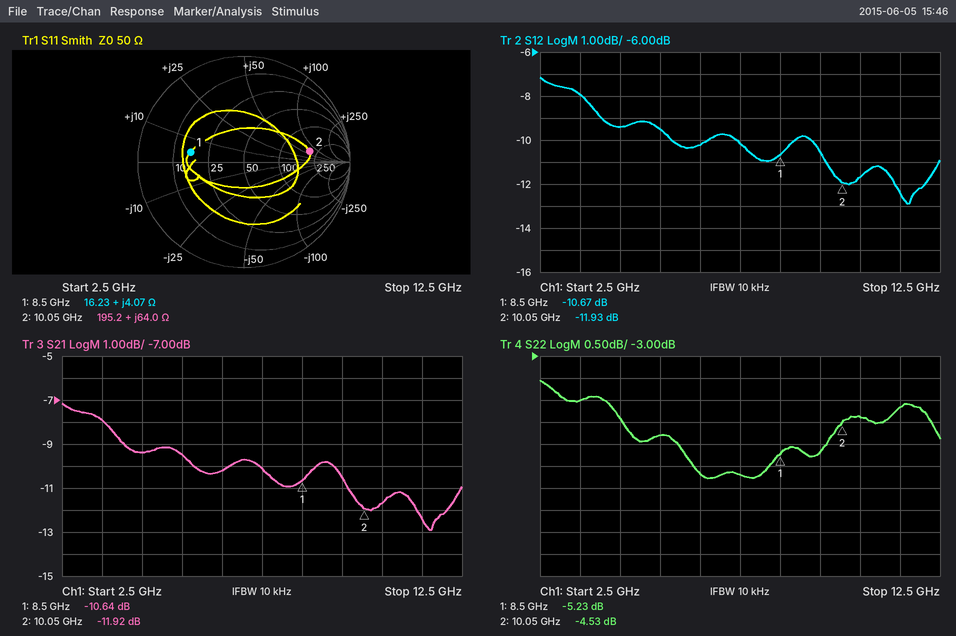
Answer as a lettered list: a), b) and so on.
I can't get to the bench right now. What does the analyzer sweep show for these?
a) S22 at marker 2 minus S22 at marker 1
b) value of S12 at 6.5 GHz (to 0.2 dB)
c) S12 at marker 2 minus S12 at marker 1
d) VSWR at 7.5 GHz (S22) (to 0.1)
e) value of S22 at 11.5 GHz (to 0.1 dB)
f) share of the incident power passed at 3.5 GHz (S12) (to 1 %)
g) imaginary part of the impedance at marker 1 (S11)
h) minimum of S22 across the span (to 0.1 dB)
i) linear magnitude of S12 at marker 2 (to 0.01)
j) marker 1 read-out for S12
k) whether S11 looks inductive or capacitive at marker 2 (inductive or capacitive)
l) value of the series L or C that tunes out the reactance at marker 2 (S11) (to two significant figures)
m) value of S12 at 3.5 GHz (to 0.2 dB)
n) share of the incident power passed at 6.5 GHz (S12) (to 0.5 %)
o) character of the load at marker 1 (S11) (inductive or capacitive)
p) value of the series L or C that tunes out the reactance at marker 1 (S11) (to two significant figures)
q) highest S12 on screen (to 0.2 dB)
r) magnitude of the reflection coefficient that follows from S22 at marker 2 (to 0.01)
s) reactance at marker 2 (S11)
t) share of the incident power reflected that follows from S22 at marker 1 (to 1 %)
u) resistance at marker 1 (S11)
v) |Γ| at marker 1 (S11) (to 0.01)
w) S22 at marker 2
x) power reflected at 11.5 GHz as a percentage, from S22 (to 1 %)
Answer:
a) 0.70 dB
b) -10.2 dB
c) -1.26 dB
d) 3.2
e) -4.2 dB
f) 16 %
g) +4.07 Ω
h) -5.8 dB
i) 0.25
j) -10.67 dB
k) inductive
l) 250 fF
m) -8.0 dB
n) 9.5 %
o) inductive
p) 4.6 pF
q) -7.2 dB
r) 0.59
s) +64.0 Ω
t) 30 %
u) 16.23 Ω
v) 0.51
w) -4.53 dB
x) 38 %
